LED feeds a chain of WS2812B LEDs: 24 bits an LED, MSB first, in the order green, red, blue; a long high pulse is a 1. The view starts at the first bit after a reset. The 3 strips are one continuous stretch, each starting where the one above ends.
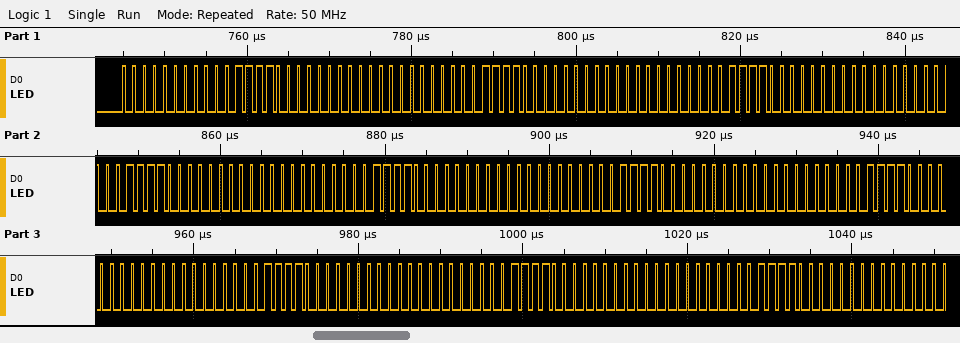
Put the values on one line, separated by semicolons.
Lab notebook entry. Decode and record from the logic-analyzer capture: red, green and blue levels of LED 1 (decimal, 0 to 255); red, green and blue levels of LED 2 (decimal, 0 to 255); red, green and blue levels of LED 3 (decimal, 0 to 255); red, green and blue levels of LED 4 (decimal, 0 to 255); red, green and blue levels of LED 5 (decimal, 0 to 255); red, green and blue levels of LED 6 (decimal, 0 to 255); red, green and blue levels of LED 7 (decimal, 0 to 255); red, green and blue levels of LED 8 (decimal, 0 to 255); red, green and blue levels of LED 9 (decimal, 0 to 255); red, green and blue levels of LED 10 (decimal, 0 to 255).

30, 0, 0; 30, 0, 0; 30, 0, 0; 30, 0, 0; 30, 0, 0; 30, 0, 0; 30, 0, 0; 30, 0, 0; 30, 0, 0; 30, 0, 0
